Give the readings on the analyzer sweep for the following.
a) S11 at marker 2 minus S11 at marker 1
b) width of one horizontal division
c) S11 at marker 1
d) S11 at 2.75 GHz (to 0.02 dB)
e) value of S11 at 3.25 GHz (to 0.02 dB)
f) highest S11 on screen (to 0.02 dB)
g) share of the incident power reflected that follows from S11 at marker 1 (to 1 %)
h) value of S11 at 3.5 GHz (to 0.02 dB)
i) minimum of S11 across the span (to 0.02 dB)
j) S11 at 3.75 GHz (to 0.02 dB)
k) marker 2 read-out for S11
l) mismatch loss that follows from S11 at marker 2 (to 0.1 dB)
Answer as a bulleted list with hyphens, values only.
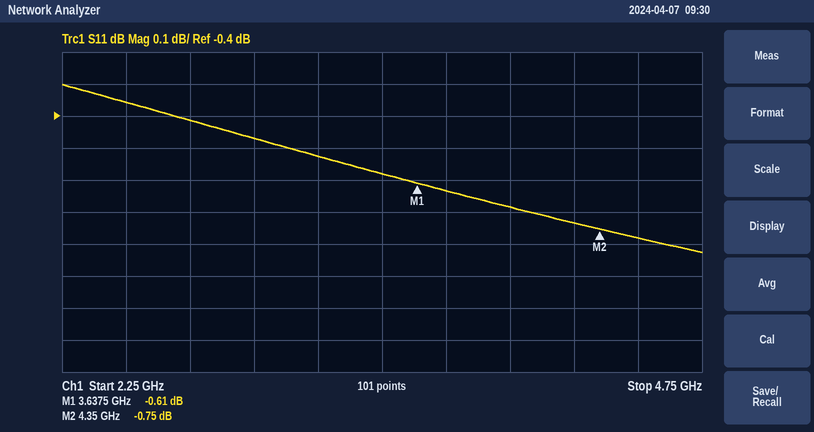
- -0.14 dB
- 250 MHz
- -0.61 dB
- -0.42 dB
- -0.52 dB
- -0.30 dB
- 87 %
- -0.58 dB
- -0.82 dB
- -0.64 dB
- -0.75 dB
- 8.0 dB
